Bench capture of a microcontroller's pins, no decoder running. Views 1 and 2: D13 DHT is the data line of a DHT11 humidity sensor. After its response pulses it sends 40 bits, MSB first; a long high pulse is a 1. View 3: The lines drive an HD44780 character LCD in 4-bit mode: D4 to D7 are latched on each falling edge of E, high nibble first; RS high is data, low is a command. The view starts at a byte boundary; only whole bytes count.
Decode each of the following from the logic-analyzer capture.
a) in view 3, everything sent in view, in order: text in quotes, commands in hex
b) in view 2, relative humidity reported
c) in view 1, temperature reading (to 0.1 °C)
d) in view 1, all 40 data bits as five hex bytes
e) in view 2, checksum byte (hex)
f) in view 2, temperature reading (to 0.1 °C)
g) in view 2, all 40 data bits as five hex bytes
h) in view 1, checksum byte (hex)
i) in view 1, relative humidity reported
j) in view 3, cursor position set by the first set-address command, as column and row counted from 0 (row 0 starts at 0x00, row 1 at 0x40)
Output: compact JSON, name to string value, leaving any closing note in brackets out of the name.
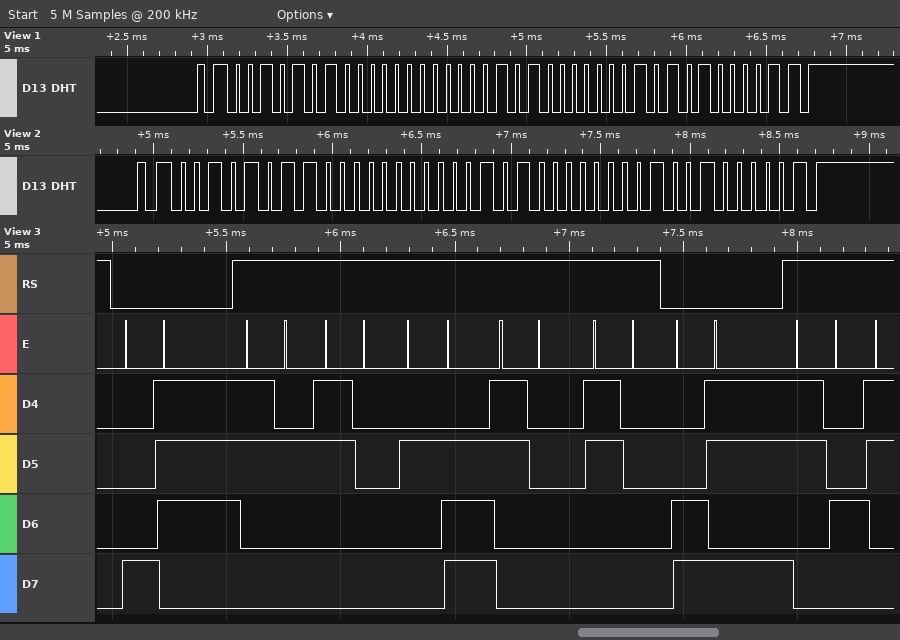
{"in view 3, everything sent in view, in order: text in quotes, commands in hex": "0x87 \"20.00\" 0xCB \"4\"", "in view 2, relative humidity reported": "43 %", "in view 1, temperature reading": "20.5 °C", "in view 1, all 40 data bits as five hex bytes": "2A 00 14 05 43", "in view 2, checksum byte": "0x41", "in view 2, temperature reading": "20.2 °C", "in view 2, all 40 data bits as five hex bytes": "2B 00 14 02 41", "in view 1, checksum byte": "0x43", "in view 1, relative humidity reported": "42 %", "in view 3, cursor position set by the first set-address command, as column and row counted from 0": "column 7, row 0"}
